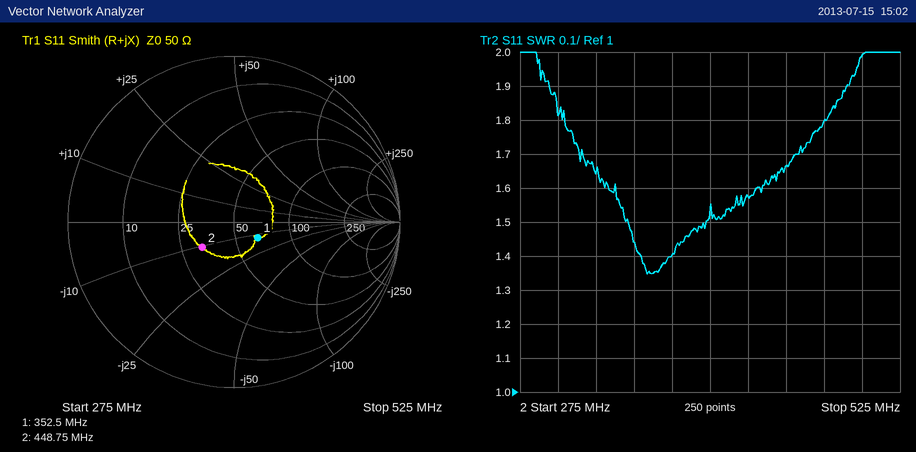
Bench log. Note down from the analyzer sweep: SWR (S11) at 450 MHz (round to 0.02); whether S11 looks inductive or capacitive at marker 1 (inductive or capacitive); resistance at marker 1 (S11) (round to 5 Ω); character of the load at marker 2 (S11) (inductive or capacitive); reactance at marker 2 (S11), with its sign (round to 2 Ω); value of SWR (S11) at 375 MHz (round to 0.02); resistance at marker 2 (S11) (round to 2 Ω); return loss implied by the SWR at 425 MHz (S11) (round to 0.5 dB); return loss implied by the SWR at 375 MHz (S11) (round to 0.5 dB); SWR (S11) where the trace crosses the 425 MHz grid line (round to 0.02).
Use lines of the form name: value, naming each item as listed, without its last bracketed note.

SWR (S11) at 450 MHz: 1.66
whether S11 looks inductive or capacitive at marker 1: capacitive
resistance at marker 1 (S11): 65 Ω
character of the load at marker 2 (S11): capacitive
reactance at marker 2 (S11), with its sign: -10 Ω
value of SWR (S11) at 375 MHz: 1.40
resistance at marker 2 (S11): 32 Ω
return loss implied by the SWR at 425 MHz (S11): 13.0 dB
return loss implied by the SWR at 375 MHz (S11): 15.5 dB
SWR (S11) where the trace crosses the 425 MHz grid line: 1.58
